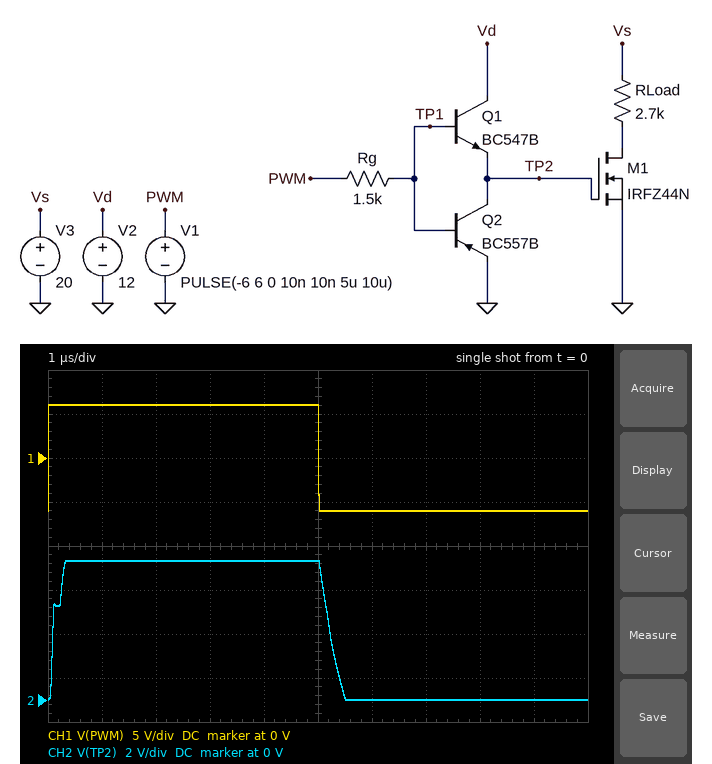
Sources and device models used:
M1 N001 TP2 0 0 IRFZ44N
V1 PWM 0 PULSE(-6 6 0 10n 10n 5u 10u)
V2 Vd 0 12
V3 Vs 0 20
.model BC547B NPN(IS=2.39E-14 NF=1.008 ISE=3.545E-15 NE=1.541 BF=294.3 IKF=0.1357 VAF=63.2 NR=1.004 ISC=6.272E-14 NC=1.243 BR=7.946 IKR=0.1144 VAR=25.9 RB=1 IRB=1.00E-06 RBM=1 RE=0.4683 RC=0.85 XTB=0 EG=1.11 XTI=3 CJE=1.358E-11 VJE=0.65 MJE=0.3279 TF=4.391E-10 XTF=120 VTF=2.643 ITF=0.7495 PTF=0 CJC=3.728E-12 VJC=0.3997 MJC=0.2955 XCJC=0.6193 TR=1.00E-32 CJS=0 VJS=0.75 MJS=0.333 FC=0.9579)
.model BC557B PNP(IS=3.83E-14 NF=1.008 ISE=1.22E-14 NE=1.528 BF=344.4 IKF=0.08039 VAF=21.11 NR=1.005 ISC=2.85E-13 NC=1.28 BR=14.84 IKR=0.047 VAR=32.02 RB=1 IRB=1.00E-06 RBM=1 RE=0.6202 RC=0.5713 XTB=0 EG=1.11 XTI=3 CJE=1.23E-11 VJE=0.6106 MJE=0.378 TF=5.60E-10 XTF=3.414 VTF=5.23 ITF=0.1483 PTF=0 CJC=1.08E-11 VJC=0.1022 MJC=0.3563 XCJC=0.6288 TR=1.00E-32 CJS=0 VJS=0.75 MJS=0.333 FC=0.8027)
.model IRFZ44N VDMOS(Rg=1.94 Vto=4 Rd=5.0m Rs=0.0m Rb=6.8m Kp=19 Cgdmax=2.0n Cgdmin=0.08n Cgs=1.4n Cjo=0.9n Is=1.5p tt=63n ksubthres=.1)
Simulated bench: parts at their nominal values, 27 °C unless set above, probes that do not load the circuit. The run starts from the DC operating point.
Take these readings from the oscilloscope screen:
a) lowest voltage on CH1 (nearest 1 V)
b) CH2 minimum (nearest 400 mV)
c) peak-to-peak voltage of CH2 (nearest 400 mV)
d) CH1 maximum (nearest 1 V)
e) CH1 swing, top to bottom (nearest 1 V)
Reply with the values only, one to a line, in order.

-6 V
0 V
6.4 V
6 V
12 V
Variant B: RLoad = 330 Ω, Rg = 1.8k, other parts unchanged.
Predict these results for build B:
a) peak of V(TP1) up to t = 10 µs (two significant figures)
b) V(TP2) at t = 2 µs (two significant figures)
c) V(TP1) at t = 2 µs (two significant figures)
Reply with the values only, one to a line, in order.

6.9 V
6.2 V
6.0 V
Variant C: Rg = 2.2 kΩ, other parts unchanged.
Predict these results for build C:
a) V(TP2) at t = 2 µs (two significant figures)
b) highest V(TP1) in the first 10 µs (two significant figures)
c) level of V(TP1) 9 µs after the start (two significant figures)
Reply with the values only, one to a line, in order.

6.1 V
6.8 V
-720 mV
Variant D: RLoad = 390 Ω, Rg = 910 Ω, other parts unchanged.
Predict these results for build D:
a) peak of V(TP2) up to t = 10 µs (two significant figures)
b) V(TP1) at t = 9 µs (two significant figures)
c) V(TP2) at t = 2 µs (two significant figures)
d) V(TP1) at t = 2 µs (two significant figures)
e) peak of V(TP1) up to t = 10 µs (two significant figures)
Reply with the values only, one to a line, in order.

6.6 V
-750 mV
6.5 V
6.0 V
7.3 V
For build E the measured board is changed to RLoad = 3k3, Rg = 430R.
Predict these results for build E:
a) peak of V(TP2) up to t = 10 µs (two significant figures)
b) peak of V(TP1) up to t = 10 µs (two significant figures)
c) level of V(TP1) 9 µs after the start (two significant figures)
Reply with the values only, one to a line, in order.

6.9 V
7.7 V
-780 mV
